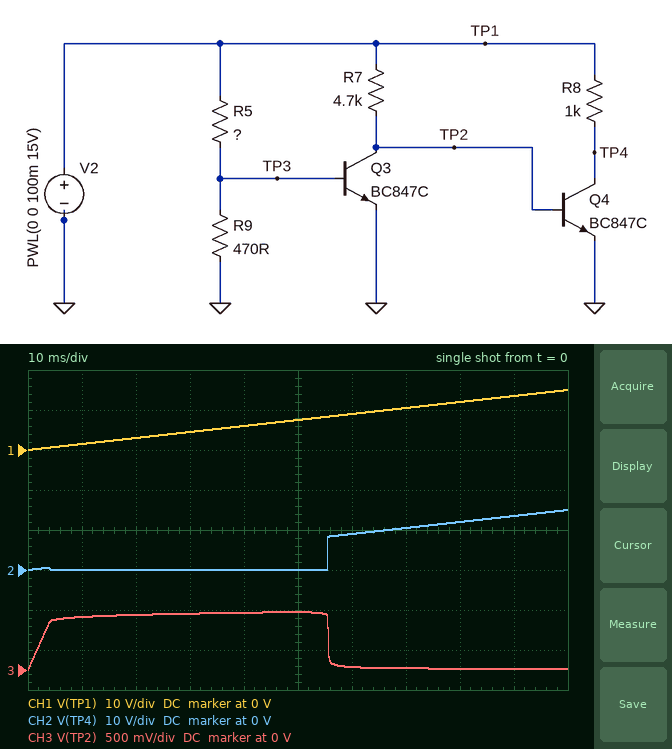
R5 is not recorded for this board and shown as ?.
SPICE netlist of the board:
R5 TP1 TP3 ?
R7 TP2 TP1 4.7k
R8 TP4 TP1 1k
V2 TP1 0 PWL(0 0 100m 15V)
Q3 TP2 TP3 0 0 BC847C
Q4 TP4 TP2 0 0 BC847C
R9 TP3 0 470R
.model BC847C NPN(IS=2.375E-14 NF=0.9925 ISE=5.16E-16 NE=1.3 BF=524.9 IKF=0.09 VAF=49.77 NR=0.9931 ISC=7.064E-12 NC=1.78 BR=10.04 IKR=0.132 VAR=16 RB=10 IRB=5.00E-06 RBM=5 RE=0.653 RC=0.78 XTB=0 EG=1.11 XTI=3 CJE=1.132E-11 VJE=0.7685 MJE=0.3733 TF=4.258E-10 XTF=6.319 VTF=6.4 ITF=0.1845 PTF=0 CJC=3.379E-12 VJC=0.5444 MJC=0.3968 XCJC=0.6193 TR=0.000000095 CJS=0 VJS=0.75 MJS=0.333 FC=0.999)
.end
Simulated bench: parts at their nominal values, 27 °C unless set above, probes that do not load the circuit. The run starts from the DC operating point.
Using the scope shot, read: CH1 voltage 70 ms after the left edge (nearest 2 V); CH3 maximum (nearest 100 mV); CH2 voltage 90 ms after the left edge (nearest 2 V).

10 V
700 mV
14 V
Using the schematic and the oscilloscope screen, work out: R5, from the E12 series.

5.6 kΩ
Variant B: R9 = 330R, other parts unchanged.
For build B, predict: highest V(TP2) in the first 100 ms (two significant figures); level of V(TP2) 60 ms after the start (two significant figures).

740 mV
730 mV
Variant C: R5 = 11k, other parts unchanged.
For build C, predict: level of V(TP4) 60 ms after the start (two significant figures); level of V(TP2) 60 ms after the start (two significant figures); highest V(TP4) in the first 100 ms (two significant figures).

30 mV
730 mV
510 mV
